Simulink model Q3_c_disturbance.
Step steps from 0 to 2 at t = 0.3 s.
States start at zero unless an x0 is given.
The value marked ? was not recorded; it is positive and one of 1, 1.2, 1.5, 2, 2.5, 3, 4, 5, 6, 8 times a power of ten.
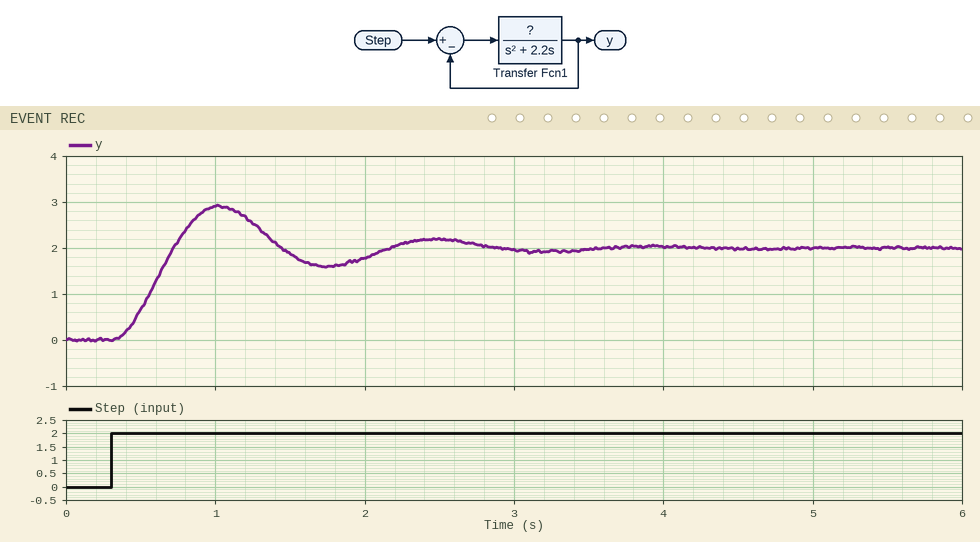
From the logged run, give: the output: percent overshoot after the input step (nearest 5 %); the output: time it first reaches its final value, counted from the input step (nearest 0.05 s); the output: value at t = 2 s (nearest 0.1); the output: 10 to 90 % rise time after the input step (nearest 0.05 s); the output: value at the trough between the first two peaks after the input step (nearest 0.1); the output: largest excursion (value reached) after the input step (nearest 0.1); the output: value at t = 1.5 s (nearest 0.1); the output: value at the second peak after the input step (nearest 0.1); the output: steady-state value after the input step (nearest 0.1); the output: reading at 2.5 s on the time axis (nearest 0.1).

45 %
0.40 s
1.8
0.30 s
1.6
2.9
1.9
2.2
2.0
2.2
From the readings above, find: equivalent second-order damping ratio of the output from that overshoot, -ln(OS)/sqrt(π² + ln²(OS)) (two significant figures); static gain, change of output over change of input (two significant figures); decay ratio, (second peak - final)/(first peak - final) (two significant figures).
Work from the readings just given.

0.25
1.0
0.22
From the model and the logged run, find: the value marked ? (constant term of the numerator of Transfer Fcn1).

20
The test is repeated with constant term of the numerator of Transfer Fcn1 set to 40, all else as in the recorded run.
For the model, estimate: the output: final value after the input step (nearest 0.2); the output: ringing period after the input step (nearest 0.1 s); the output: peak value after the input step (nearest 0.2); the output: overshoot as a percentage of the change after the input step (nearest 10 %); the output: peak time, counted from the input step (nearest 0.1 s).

2.0
1.0 s
3.2
60 %
0.5 s
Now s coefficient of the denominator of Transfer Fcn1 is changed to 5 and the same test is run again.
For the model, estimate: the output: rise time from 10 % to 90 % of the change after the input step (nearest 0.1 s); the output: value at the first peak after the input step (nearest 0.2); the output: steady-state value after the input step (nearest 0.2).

0.4 s
2.2
2.0
